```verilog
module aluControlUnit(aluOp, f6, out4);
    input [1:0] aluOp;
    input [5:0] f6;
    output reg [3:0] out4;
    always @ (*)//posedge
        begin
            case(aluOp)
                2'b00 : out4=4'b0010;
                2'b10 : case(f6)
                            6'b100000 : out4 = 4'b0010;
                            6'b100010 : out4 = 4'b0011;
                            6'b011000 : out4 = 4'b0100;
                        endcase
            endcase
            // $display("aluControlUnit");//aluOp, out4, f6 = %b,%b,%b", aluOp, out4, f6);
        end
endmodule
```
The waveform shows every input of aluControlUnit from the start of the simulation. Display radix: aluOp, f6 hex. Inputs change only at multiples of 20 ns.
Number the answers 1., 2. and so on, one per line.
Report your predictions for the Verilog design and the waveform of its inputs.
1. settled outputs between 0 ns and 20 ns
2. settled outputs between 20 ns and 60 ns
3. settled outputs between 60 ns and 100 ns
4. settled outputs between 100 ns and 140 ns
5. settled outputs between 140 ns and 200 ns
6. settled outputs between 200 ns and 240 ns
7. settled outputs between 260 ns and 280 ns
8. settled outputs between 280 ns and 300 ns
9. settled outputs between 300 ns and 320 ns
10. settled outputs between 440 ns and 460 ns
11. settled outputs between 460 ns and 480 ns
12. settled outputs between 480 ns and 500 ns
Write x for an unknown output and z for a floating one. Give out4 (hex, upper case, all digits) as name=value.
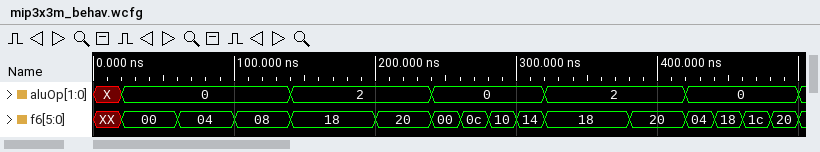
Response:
1. out4=x
2. out4=2
3. out4=2
4. out4=2
5. out4=4
6. out4=2
7. out4=2
8. out4=2
9. out4=2
10. out4=2
11. out4=2
12. out4=2
